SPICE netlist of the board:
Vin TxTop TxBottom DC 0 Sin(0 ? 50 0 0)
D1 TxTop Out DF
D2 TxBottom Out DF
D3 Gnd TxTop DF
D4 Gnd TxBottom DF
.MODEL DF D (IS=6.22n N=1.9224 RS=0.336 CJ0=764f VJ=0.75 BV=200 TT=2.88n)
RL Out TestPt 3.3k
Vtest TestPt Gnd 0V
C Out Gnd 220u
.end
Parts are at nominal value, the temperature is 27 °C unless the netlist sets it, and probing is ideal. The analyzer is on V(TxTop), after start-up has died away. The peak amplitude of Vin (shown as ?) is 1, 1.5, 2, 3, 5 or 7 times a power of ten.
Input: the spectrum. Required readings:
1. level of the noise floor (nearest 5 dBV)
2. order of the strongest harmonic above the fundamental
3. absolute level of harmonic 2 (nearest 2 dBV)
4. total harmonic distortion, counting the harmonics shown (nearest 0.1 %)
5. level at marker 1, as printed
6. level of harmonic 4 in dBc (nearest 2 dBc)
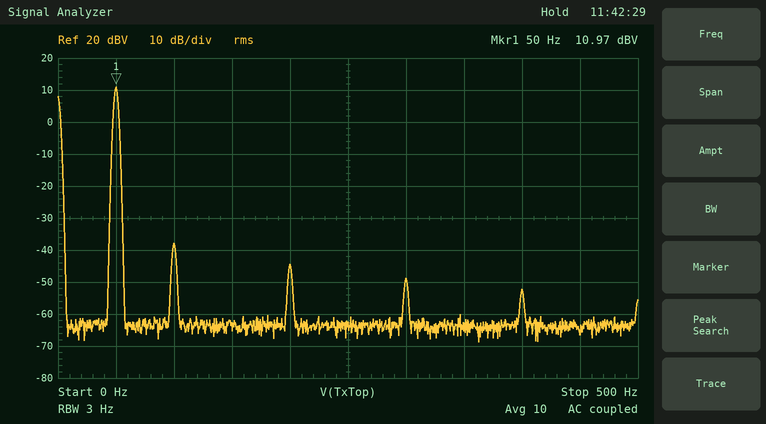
-65 dBV
2
-38 dBV
0.4 %
10.97 dBV
-56 dBc
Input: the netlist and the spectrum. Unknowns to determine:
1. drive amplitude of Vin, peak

10 V
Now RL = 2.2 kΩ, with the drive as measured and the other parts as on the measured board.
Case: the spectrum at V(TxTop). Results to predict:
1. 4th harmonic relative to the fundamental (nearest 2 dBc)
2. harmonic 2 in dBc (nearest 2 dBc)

-52 dBc
-46 dBc
